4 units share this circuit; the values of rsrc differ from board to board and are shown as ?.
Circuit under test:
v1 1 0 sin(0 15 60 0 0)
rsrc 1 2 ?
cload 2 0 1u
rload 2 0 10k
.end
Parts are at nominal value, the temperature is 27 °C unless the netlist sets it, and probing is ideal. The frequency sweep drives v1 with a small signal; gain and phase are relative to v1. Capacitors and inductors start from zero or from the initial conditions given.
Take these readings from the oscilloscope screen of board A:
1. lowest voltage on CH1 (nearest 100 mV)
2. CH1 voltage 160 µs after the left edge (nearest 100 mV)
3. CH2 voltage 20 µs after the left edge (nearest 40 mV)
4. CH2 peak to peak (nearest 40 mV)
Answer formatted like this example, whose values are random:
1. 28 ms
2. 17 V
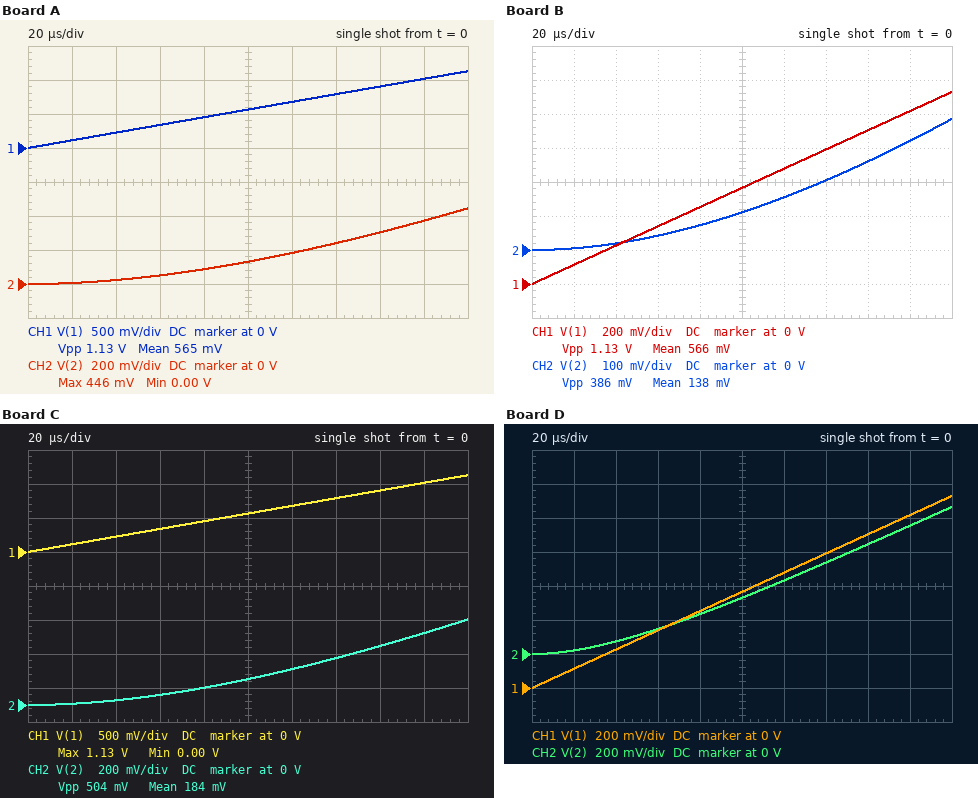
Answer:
1. 0 V
2. 900 mV
3. 0 V
4. 440 mV
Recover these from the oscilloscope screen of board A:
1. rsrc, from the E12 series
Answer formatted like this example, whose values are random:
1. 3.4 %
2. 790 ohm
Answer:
1. 180 Ω
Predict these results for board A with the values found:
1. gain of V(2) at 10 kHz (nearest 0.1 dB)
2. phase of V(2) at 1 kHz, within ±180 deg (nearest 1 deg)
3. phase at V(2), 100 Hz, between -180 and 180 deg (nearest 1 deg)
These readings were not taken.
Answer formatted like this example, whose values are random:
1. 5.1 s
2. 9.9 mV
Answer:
1. -21.1 dB
2. -48 deg
3. -6 deg
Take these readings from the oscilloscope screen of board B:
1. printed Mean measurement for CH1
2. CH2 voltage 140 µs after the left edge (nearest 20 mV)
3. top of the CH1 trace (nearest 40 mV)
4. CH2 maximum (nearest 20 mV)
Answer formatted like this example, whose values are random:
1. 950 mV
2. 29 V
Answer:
1. 566 mV
2. 200 mV
3. 1.12 V
4. 380 mV
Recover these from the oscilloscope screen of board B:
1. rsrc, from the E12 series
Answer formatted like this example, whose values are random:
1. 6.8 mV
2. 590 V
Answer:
1. 220 Ω
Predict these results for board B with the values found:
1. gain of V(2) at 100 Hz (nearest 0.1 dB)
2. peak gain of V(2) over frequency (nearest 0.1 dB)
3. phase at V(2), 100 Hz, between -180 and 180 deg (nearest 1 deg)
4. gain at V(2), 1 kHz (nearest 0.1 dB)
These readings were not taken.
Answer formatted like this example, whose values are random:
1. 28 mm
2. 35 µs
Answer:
1. -0.3 dB
2. -0.2 dB
3. -8 deg
4. -4.7 dB
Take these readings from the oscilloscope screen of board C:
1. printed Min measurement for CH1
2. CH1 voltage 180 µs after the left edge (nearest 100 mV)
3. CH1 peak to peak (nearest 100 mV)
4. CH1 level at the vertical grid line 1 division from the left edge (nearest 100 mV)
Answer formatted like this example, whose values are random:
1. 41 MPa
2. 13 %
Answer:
1. 0.00 V
2. 1.0 V
3. 1.1 V
4. 100 mV
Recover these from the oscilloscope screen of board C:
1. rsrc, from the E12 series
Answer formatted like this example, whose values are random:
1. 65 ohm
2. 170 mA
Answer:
1. 150 Ω
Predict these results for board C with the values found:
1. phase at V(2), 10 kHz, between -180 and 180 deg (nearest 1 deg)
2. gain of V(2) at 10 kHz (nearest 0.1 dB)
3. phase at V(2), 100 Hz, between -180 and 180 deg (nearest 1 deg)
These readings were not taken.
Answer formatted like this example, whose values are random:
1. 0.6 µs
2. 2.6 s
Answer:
1. -84 deg
2. -19.5 dB
3. -5 deg
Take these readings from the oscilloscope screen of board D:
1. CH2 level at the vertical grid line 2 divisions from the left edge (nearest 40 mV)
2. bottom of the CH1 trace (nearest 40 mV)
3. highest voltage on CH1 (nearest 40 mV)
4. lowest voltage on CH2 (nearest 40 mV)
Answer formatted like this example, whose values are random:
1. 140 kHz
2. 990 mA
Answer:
1. 80 mV
2. 0 V
3. 1.12 V
4. 0 V
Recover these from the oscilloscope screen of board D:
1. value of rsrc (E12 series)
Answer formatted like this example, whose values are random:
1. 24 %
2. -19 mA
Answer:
1. 47 Ω
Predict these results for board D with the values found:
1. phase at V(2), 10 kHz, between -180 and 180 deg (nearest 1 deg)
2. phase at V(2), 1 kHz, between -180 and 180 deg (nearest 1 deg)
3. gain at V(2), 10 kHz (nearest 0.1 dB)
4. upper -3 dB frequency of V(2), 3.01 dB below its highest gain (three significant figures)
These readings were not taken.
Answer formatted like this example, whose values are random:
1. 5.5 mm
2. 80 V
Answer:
1. -71 deg
2. -16 deg
3. -9.9 dB
4. 3.40 kHz
